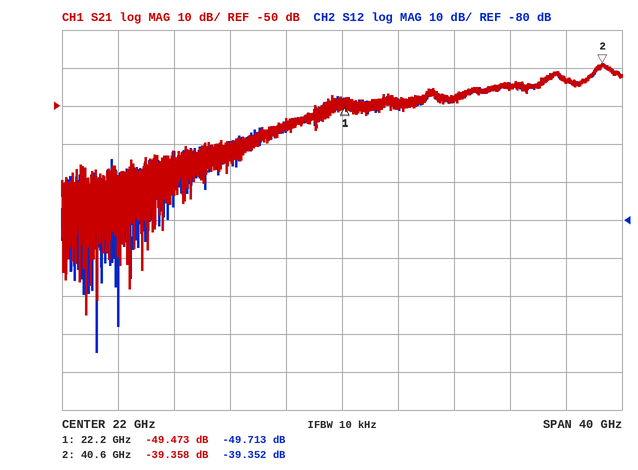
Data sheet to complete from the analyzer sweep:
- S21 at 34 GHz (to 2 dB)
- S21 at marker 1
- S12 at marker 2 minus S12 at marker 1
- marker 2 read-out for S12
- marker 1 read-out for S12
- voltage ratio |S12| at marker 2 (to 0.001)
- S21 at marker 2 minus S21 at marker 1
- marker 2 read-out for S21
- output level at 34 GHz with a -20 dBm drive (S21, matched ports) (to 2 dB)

-44 dB
-49.473 dB
10.361 dB
-39.352 dB
-49.713 dB
0.011
10.115 dB
-39.358 dB
-64 dBm
